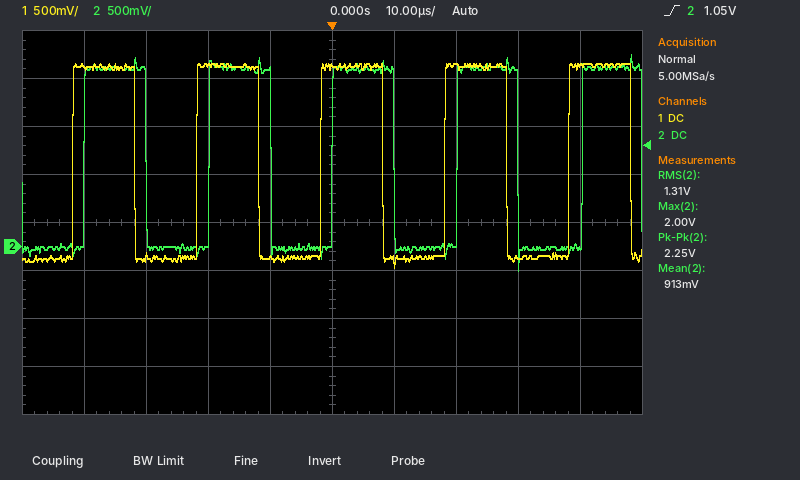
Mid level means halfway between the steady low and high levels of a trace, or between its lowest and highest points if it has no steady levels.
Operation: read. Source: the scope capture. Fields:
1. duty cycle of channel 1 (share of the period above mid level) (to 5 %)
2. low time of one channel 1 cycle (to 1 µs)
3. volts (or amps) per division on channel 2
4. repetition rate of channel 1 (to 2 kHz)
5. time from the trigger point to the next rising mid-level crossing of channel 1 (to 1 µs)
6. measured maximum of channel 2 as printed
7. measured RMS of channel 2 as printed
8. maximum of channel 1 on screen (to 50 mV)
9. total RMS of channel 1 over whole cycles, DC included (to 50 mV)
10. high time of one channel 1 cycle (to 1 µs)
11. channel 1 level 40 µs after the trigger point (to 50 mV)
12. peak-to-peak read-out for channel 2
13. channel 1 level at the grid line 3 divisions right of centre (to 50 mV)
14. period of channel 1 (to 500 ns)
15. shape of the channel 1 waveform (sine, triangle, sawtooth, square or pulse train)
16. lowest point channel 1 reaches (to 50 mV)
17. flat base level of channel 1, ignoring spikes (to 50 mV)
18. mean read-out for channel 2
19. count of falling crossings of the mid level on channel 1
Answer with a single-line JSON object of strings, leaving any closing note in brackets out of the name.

{"duty cycle of channel 1 (share of the period above mid level)": "50 %", "low time of one channel 1 cycle": "10 µs", "volts (or amps) per division on channel 2": "500 mV", "repetition rate of channel 1": "50 kHz", "time from the trigger point to the next rising mid-level crossing of channel 1": "18 µs", "measured maximum of channel 2 as printed": "2.00 V", "measured RMS of channel 2 as printed": "1.31 V", "maximum of channel 1 on screen": "1.90 V", "total RMS of channel 1 over whole cycles, DC included": "1.35 V", "high time of one channel 1 cycle": "10 µs", "channel 1 level 40 µs after the trigger point": "1.90 V", "peak-to-peak read-out for channel 2": "2.25 V", "channel 1 level at the grid line 3 divisions right of centre": "-100 mV", "period of channel 1": "20.0 µs", "shape of the channel 1 waveform": "square", "lowest point channel 1 reaches": "-200 mV", "flat base level of channel 1, ignoring spikes": "-100 mV", "mean read-out for channel 2": "913 mV", "count of falling crossings of the mid level on channel 1": "5"}
